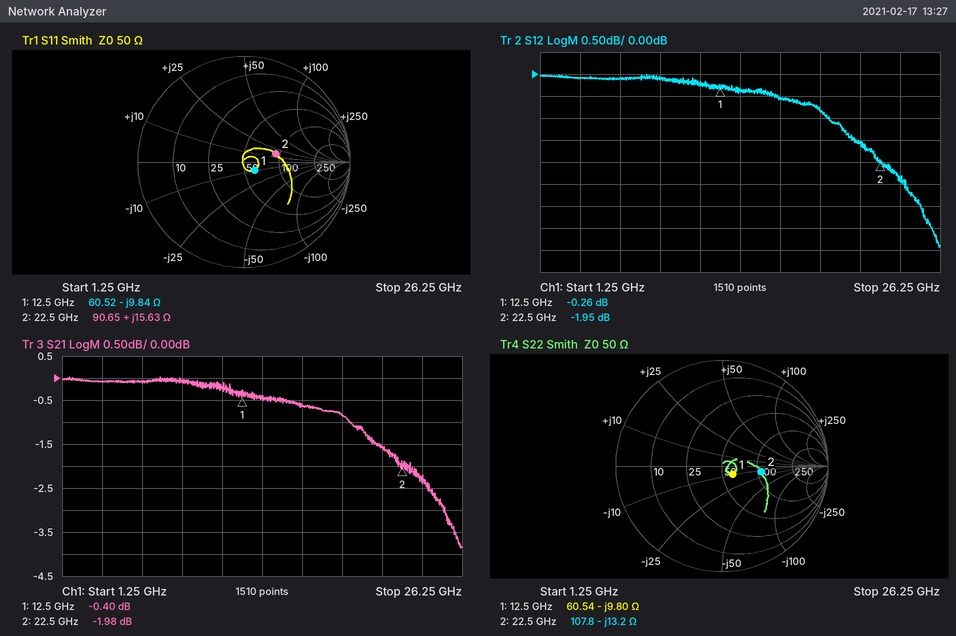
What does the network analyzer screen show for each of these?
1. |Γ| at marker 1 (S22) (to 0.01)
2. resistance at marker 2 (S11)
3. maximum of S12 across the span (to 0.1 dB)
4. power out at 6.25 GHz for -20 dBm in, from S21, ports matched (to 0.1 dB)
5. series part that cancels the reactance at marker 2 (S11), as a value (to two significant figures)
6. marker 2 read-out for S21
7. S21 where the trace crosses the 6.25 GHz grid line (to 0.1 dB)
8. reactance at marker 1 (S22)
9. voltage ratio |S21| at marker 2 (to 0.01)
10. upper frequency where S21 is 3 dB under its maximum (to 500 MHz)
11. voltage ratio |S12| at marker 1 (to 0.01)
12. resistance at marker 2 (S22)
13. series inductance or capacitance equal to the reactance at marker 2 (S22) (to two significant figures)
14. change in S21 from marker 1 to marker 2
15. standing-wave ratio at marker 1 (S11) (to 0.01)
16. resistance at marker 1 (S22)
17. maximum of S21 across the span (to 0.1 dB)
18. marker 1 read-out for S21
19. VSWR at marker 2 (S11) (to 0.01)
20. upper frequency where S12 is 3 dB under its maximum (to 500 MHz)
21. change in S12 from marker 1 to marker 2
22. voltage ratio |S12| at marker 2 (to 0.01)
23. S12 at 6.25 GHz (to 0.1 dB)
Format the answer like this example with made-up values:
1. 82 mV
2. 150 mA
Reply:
1. 0.13
2. 90.65 Ω
3. 0.0 dB
4. -20.1 dBm
5. 450 fF
6. -1.98 dB
7. -0.1 dB
8. -9.80 Ω
9. 0.80
10. 25.0 GHz
11. 0.97
12. 107.8 Ω
13. 540 fF
14. -1.58 dB
15. 1.30
16. 60.54 Ω
17. 0.0 dB
18. -0.40 dB
19. 1.89
20. 25.0 GHz
21. -1.69 dB
22. 0.80
23. -0.1 dB
